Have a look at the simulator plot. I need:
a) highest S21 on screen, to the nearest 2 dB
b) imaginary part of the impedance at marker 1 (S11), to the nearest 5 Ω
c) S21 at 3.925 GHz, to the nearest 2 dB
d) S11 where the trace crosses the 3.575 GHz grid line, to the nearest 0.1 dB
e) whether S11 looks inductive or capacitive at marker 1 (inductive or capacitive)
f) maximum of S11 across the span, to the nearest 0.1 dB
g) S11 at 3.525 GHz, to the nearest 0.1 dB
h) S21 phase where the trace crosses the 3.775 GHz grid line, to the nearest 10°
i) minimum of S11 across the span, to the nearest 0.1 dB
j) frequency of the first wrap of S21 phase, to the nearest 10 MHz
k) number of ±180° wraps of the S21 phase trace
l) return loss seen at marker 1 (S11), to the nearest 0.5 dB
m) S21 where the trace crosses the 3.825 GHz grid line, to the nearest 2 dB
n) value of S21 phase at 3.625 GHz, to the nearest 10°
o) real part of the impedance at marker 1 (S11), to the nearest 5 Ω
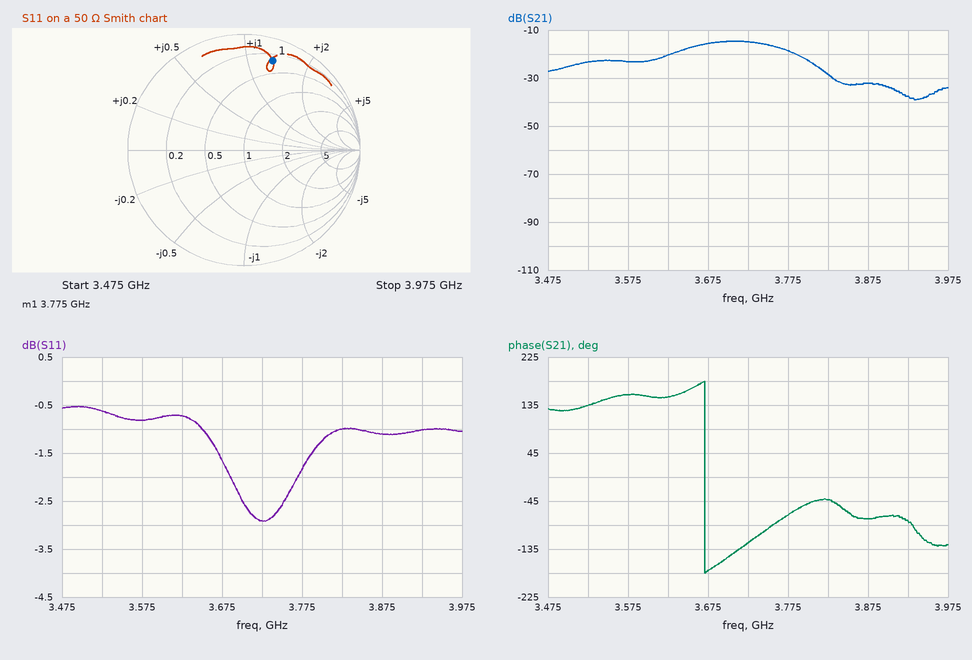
-14 dB
+65 Ω
-38 dB
-0.8 dB
inductive
-0.5 dB
-0.6 dB
-70°
-2.9 dB
3.67 GHz
1
2.0 dB
-28 dB
150°
15 Ω
